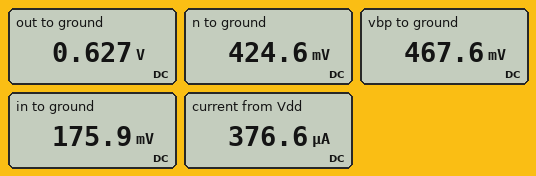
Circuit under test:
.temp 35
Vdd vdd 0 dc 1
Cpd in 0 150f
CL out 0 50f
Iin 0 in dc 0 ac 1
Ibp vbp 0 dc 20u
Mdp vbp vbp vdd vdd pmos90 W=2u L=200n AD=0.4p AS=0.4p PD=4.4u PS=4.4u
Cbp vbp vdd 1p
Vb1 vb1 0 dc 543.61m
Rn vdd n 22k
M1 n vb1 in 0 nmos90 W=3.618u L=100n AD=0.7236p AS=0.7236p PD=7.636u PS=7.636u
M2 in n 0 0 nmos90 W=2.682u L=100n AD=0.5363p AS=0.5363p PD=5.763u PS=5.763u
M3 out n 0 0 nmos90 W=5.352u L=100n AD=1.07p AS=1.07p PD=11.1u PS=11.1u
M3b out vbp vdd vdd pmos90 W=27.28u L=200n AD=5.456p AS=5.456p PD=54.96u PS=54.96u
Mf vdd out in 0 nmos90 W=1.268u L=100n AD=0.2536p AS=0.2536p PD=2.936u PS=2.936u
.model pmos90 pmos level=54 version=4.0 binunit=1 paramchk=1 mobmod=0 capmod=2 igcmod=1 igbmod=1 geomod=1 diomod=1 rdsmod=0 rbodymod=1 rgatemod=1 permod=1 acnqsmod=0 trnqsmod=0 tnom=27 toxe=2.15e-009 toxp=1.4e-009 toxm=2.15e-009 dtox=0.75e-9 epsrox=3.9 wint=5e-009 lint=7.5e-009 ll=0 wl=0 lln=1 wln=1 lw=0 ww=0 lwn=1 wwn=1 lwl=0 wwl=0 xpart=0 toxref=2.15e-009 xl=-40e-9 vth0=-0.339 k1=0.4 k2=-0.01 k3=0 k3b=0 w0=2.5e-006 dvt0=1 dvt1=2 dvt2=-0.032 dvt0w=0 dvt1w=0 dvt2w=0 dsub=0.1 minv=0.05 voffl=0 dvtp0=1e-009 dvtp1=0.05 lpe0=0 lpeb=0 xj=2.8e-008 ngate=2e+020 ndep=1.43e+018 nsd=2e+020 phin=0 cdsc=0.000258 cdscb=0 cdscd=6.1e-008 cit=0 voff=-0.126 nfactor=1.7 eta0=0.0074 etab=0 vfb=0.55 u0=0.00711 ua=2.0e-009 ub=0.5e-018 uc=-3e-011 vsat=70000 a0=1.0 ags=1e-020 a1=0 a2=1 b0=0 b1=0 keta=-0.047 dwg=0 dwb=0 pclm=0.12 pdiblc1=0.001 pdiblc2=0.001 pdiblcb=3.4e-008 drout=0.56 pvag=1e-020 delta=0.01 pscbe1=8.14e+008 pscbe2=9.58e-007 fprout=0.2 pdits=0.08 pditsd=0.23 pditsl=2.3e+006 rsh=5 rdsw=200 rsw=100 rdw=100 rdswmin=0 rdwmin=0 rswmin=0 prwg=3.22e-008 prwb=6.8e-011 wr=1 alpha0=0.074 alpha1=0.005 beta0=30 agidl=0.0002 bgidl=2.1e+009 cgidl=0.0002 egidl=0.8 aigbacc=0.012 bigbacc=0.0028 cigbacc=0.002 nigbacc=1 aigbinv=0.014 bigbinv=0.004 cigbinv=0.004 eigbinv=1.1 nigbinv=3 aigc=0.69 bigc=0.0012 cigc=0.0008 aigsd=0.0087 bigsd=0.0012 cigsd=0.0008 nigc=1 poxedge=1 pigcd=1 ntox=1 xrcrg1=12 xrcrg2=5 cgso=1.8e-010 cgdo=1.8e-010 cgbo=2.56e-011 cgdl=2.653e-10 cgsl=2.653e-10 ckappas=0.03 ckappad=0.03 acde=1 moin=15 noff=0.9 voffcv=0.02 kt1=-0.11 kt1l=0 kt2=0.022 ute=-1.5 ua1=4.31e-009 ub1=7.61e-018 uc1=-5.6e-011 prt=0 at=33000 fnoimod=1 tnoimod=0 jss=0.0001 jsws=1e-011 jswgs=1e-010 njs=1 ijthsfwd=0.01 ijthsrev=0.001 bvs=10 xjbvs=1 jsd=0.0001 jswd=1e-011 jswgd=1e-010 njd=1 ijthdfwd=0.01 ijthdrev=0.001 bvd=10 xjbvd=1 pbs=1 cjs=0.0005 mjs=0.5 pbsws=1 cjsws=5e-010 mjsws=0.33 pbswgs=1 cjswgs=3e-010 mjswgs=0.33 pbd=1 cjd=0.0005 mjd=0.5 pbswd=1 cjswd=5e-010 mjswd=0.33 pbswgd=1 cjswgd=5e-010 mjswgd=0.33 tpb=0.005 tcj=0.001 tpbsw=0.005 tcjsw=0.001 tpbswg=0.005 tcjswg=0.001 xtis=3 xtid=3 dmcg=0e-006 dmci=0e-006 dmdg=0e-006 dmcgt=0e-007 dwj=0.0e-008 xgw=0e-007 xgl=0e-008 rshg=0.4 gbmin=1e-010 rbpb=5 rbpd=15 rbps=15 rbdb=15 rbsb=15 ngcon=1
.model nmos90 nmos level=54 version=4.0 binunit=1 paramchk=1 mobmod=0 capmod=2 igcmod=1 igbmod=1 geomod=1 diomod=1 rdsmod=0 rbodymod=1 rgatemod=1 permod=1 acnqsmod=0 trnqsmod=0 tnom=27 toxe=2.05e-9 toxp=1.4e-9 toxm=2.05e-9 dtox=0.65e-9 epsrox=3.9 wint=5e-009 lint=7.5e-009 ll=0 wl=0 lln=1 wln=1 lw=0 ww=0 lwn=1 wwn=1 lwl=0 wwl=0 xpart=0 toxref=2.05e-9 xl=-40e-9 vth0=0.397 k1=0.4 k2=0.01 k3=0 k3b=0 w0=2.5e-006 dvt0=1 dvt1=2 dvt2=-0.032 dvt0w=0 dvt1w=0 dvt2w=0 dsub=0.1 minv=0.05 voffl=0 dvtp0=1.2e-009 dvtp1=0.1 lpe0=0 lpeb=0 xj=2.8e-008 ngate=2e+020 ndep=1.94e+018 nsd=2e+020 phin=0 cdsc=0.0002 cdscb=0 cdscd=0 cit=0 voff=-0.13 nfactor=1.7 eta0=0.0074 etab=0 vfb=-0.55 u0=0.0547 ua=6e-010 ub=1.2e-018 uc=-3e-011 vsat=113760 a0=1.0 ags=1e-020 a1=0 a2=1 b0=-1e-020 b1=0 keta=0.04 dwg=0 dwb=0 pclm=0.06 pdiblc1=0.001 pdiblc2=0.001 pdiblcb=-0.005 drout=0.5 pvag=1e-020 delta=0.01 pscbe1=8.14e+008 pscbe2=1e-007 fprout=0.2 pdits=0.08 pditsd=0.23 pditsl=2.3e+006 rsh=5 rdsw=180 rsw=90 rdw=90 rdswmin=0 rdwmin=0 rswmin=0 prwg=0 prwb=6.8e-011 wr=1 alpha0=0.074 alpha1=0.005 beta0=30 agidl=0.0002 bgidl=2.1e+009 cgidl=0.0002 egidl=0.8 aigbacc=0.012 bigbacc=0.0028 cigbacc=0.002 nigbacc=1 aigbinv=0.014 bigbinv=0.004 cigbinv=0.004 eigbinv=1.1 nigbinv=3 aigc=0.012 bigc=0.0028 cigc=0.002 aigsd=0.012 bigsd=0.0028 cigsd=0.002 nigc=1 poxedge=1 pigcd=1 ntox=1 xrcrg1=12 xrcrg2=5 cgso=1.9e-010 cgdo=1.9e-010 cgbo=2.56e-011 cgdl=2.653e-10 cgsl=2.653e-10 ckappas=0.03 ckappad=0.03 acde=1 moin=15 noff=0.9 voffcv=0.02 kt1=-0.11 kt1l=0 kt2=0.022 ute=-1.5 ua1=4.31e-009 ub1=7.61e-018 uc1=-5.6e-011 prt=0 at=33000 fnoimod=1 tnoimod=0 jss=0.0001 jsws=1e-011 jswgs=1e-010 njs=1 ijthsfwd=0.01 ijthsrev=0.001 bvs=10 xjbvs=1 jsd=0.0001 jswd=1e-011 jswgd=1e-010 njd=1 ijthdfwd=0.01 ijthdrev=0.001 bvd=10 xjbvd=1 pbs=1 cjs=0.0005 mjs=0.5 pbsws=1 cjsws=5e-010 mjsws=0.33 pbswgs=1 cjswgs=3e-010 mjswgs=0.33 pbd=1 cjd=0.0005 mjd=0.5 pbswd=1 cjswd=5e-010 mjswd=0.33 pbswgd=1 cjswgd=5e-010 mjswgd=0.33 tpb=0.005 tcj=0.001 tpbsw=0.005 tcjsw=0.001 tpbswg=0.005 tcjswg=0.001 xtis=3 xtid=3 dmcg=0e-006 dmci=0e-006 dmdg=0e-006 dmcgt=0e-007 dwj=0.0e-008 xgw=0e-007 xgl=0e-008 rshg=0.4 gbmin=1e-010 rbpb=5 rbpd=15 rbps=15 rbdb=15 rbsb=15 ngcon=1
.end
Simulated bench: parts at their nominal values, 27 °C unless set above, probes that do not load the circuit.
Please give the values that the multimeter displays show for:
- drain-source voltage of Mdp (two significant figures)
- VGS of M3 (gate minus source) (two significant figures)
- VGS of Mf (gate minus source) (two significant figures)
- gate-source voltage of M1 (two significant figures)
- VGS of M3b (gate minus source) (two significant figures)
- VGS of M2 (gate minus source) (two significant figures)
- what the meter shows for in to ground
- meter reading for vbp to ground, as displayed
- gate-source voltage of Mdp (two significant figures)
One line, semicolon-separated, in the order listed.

-530 mV; 420 mV; 450 mV; 370 mV; -530 mV; 420 mV; 175.9 mV; 467.6 mV; -530 mV
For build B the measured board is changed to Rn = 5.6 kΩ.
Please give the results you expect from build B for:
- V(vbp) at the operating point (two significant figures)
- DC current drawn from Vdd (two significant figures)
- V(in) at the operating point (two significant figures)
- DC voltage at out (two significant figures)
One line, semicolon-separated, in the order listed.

470 mV; 400 µA; 120 mV; 390 mV
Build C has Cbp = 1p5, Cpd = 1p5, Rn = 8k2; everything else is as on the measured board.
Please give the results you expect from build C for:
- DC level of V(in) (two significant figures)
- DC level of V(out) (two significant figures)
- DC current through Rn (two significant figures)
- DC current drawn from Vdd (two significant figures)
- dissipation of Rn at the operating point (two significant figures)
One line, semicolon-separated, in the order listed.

130 mV; 510 mV; 69 µA; 390 µA; 39 µW
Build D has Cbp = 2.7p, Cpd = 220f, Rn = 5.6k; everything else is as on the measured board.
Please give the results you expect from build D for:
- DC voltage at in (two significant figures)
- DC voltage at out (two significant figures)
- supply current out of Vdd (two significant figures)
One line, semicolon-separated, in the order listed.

120 mV; 390 mV; 400 µA
